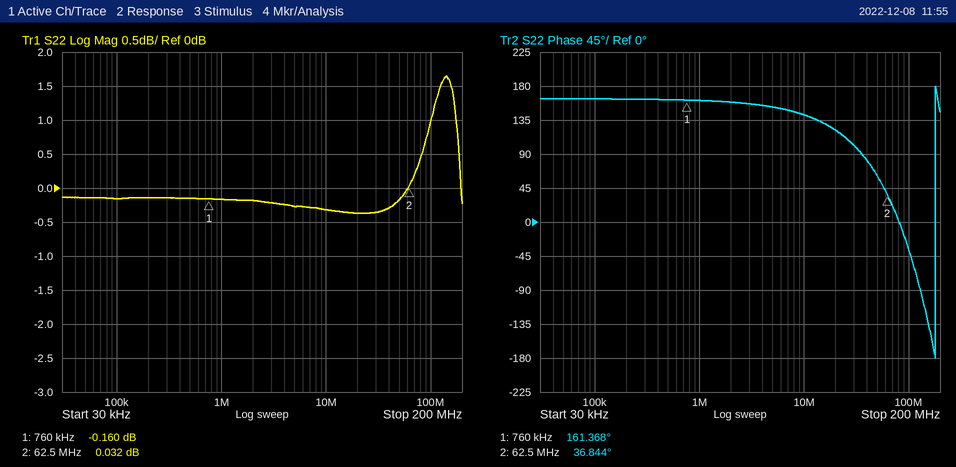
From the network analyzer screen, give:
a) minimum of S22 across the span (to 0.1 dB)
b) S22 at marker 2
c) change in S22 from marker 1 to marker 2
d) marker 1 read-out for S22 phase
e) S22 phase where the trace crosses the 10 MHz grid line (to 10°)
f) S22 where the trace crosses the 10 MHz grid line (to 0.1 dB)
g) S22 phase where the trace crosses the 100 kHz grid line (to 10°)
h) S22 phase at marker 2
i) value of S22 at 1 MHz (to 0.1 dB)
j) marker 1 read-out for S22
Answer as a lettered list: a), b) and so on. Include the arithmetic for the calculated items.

a) -0.4 dB
b) 0.032 dB
c) 0.032 − (-0.16) = 0.192 dB
d) 161.368°
e) 140°
f) -0.3 dB
g) 160°
h) 36.844°
i) -0.2 dB
j) -0.160 dB
